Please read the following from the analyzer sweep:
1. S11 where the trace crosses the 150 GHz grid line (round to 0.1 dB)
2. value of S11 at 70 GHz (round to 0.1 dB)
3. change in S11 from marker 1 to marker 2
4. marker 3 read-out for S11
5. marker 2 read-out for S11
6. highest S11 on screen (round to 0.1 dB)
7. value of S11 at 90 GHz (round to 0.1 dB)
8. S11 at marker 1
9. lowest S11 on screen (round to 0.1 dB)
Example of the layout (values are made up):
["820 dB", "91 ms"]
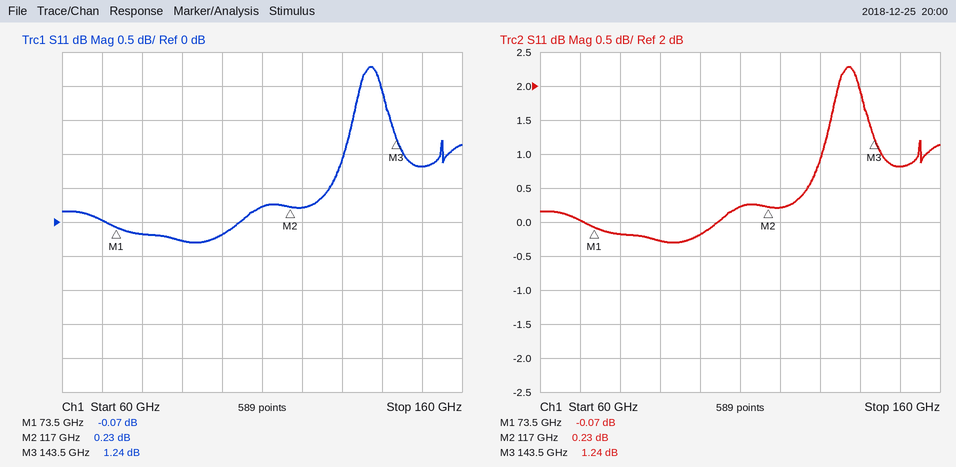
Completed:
["0.8 dB", "0.0 dB", "0.30 dB", "1.24 dB", "0.23 dB", "2.3 dB", "-0.3 dB", "-0.07 dB", "-0.3 dB"]
